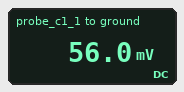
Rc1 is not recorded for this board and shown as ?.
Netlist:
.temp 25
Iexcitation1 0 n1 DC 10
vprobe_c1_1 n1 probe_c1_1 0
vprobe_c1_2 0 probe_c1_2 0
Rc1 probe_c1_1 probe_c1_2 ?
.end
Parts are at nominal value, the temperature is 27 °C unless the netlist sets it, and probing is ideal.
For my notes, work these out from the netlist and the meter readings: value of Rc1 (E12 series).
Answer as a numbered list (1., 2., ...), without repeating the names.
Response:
1. 5.6 mΩ
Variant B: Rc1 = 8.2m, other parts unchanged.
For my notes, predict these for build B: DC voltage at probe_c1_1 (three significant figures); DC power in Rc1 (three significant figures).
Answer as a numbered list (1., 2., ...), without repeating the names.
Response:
1. 82.0 mV
2. 820 mW
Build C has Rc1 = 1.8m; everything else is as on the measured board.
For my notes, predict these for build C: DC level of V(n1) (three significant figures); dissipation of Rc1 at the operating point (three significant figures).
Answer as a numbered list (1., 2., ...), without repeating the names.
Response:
1. 18.0 mV
2. 180 mW
